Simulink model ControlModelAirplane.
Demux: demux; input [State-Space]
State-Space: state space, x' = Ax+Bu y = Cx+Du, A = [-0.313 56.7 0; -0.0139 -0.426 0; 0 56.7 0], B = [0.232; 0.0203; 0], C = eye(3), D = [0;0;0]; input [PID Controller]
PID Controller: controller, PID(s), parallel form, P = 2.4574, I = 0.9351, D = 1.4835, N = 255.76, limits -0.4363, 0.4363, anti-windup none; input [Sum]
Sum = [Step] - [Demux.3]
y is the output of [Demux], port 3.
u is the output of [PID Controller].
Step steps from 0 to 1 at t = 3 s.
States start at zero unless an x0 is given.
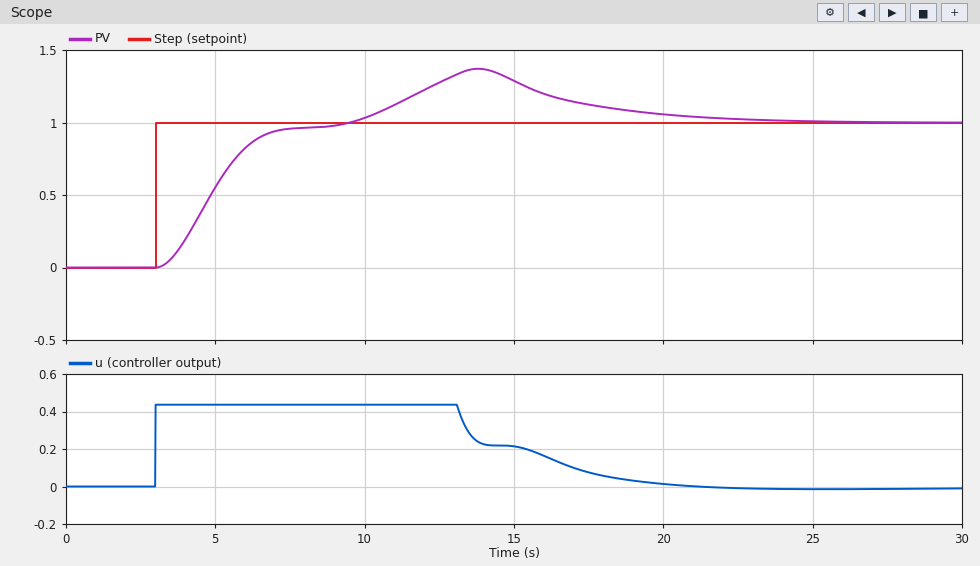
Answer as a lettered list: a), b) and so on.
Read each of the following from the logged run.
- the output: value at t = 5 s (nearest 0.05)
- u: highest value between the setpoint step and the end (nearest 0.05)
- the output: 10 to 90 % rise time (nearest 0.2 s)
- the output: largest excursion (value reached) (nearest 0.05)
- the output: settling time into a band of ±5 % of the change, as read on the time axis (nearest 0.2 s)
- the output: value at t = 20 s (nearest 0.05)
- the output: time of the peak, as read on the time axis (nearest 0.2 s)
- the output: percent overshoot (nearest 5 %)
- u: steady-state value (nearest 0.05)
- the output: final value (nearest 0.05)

a) 0.55
b) 0.45
c) 2.8 s
d) 1.35
e) 20.4 s
f) 1.05
g) 13.8 s
h) 35 %
i) 0.00
j) 1.00
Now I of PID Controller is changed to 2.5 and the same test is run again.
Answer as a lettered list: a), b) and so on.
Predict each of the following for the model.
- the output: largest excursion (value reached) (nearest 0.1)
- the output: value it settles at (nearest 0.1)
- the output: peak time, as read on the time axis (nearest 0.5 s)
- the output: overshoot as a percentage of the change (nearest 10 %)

a) 1.5
b) 1.0
c) 15.5 s
d) 50 %
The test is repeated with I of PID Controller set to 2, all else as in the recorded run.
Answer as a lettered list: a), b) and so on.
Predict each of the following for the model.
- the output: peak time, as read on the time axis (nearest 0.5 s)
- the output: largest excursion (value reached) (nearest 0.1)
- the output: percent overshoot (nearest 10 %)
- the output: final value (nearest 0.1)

a) 15.0 s
b) 1.5
c) 50 %
d) 1.0
